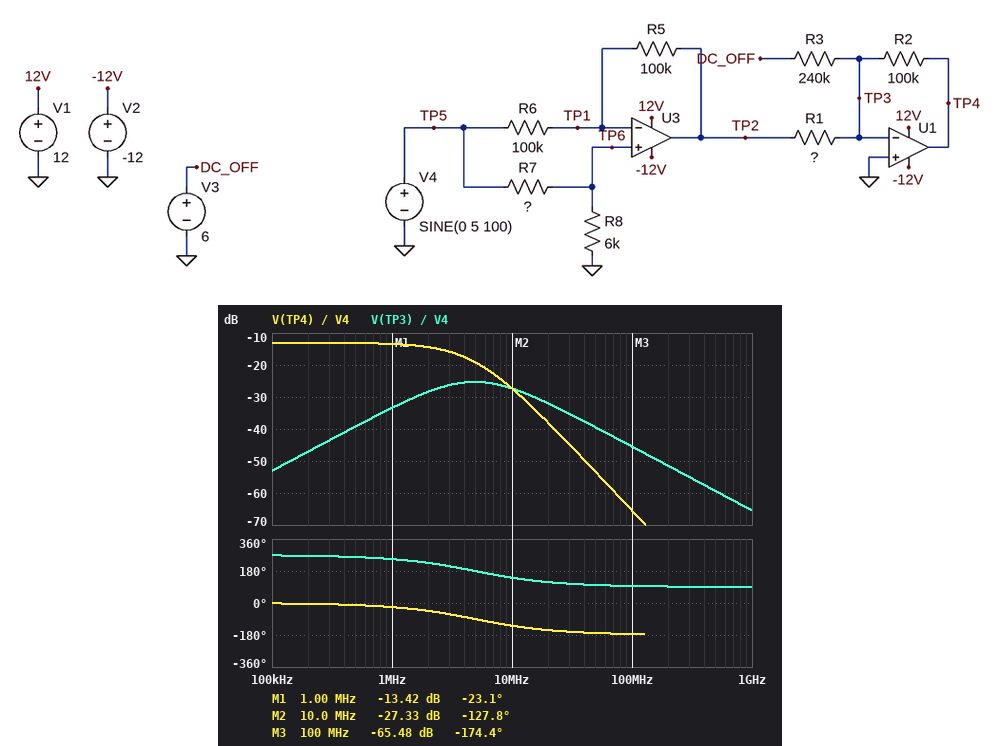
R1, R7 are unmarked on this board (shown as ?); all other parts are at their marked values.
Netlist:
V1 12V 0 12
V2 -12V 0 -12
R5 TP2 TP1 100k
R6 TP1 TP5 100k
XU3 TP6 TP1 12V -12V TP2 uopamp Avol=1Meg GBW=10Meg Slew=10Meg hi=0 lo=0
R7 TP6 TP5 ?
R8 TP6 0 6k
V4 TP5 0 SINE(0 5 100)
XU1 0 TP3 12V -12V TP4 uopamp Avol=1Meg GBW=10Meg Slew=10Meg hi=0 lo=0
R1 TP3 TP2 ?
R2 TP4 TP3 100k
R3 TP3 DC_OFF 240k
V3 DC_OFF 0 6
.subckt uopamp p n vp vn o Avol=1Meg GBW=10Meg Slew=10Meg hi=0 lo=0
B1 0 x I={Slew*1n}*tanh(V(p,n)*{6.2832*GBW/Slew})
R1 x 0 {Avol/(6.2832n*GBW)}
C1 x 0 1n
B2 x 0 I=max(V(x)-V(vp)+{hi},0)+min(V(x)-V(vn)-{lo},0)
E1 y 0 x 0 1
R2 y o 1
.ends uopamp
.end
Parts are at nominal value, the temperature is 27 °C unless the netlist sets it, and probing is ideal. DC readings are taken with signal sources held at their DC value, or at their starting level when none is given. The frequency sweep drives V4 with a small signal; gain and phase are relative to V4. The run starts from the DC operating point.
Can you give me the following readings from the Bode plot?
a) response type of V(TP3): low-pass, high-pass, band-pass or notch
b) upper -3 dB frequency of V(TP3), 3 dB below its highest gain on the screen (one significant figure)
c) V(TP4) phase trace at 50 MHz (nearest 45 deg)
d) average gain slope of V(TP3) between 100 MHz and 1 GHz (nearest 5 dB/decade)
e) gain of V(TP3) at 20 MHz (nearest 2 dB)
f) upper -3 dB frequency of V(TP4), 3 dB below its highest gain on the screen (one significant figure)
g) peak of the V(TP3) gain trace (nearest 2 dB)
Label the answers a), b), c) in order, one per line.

a) band-pass
b) 10 MHz
c) -180 deg
d) -20 dB/decade
e) -32 dB
f) 3 MHz
g) -26 dB
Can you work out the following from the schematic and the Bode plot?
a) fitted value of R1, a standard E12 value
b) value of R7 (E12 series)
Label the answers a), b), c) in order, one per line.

a) 150 kΩ
b) 12 kΩ
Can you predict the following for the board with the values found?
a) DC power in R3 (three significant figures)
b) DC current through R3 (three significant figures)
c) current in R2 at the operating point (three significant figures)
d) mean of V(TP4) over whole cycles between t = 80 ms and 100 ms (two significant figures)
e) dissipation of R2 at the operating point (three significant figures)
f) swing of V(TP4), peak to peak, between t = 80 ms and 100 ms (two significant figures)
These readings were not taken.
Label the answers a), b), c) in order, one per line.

a) 150 µW
b) 25.0 µA
c) 25.0 µA
d) -2.5 V
e) 62.5 µW
f) 2.2 V
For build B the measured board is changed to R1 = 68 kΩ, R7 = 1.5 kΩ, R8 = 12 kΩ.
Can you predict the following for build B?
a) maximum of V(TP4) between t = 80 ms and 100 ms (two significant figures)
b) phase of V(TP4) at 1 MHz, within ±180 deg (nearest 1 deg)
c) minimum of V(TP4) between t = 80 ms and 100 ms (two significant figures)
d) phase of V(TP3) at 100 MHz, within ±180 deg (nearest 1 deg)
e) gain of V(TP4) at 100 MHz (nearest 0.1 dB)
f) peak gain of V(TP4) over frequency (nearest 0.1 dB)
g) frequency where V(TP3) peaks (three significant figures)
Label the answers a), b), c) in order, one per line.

a) 3.2 V
b) 153 deg
c) -8.2 V
d) -85 deg
e) -54.1 dB
f) 1.2 dB
g) 4.16 MHz
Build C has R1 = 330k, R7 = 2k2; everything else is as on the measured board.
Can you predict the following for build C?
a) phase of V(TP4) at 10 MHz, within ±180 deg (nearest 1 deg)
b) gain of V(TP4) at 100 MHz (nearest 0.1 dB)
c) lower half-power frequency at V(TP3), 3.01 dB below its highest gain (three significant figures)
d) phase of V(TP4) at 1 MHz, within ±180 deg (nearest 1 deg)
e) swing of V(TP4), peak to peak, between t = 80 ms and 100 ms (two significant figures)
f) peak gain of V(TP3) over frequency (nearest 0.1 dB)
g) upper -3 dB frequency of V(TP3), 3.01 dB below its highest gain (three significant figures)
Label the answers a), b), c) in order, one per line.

a) 57 deg
b) -67.8 dB
c) 2.23 MHz
d) 159 deg
e) 1.4 V
f) -28.5 dB
g) 13.0 MHz
